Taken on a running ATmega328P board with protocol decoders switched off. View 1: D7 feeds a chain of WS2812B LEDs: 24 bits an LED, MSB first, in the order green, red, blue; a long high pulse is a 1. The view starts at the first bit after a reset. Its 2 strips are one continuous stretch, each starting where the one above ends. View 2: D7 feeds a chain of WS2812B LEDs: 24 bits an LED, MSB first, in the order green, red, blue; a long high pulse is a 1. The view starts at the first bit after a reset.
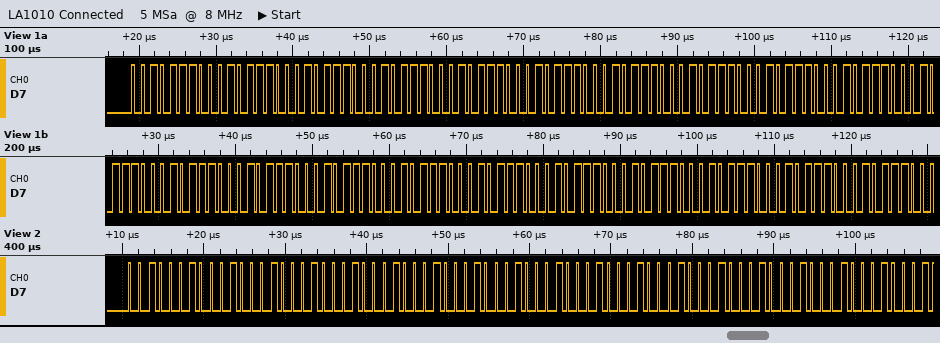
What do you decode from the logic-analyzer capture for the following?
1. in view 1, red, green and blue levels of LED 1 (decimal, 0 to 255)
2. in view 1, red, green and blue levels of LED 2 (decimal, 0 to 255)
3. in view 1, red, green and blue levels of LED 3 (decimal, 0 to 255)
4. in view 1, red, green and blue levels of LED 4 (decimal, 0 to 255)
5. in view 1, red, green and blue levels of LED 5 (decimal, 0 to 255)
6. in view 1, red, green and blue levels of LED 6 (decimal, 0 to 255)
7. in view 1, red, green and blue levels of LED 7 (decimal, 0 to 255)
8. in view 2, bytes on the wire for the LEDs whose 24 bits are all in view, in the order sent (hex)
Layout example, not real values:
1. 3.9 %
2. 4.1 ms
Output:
1. 46, 46, 46
2. 46, 46, 46
3. 46, 46, 46
4. 46, 46, 46
5. 46, 46, 46
6. 46, 46, 46
7. 46, 46, 46
8. 22 22 22 22 22 22 22 22 22
